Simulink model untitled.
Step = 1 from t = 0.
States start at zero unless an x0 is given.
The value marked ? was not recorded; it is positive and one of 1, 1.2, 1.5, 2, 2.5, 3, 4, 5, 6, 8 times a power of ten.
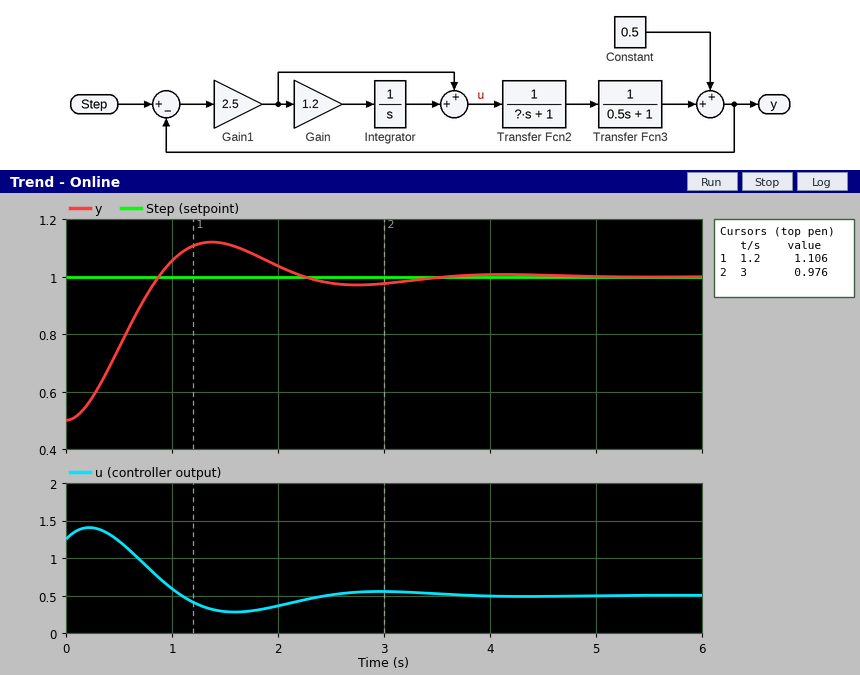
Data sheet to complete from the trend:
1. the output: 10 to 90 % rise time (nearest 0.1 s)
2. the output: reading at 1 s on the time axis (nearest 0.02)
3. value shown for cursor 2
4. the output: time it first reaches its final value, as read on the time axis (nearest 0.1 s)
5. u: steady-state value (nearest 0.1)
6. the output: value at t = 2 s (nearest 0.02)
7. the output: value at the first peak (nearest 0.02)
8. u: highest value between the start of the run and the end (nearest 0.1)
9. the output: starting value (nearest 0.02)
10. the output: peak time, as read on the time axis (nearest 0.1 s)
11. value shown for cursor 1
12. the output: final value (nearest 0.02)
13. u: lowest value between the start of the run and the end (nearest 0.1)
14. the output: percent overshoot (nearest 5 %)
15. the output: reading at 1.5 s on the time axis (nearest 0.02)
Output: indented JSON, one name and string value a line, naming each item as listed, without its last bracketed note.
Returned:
{
  "the output: 10 to 90 % rise time": "0.6 s",
  "the output: reading at 1 s on the time axis": "1.06",
  "value shown for cursor 2": "0.976",
  "the output: time it first reaches its final value, as read on the time axis": "0.9 s",
  "u: steady-state value": "0.5",
  "the output: value at t = 2 s": "1.04",
  "the output: value at the first peak": "1.12",
  "u: highest value between the start of the run and the end": "1.4",
  "the output: starting value": "0.50",
  "the output: peak time, as read on the time axis": "1.4 s",
  "value shown for cursor 1": "1.106",
  "the output: final value": "1.00",
  "u: lowest value between the start of the run and the end": "0.3",
  "the output: percent overshoot": "25 %",
  "the output: reading at 1.5 s on the time axis": "1.12"
}
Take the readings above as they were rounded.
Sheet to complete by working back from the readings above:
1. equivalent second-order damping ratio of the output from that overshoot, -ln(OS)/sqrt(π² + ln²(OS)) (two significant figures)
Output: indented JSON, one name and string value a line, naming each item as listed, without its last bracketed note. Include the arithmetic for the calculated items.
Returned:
{
  "equivalent second-order damping ratio of the output from that overshoot, -ln(OS)/sqrt(π² + ln²(OS))": "ln(0.25) = -1.386; 1.386 / sqrt(9.870 + 1.922) = 0.40"
}
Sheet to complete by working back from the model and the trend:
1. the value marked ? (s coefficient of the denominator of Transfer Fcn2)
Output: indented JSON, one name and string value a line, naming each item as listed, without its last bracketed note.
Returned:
{
  "the value marked ?": "0.8"
}
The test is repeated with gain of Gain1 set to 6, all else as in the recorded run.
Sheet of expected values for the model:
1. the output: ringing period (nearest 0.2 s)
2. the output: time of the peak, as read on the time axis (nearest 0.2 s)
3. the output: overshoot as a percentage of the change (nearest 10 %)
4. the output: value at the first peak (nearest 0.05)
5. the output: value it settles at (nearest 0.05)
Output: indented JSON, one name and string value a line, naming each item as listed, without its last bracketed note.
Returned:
{
  "the output: ringing period": "1.6 s",
  "the output: time of the peak, as read on the time axis": "0.8 s",
  "the output: overshoot as a percentage of the change": "40 %",
  "the output: value at the first peak": "1.20",
  "the output: value it settles at": "1.00"
}
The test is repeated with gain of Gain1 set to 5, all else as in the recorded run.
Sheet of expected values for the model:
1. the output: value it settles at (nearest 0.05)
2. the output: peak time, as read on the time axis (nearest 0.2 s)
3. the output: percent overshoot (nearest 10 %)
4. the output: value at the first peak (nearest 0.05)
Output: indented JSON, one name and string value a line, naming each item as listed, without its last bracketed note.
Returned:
{
  "the output: value it settles at": "1.00",
  "the output: peak time, as read on the time axis": "1.0 s",
  "the output: percent overshoot": "40 %",
  "the output: value at the first peak": "1.20"
}
